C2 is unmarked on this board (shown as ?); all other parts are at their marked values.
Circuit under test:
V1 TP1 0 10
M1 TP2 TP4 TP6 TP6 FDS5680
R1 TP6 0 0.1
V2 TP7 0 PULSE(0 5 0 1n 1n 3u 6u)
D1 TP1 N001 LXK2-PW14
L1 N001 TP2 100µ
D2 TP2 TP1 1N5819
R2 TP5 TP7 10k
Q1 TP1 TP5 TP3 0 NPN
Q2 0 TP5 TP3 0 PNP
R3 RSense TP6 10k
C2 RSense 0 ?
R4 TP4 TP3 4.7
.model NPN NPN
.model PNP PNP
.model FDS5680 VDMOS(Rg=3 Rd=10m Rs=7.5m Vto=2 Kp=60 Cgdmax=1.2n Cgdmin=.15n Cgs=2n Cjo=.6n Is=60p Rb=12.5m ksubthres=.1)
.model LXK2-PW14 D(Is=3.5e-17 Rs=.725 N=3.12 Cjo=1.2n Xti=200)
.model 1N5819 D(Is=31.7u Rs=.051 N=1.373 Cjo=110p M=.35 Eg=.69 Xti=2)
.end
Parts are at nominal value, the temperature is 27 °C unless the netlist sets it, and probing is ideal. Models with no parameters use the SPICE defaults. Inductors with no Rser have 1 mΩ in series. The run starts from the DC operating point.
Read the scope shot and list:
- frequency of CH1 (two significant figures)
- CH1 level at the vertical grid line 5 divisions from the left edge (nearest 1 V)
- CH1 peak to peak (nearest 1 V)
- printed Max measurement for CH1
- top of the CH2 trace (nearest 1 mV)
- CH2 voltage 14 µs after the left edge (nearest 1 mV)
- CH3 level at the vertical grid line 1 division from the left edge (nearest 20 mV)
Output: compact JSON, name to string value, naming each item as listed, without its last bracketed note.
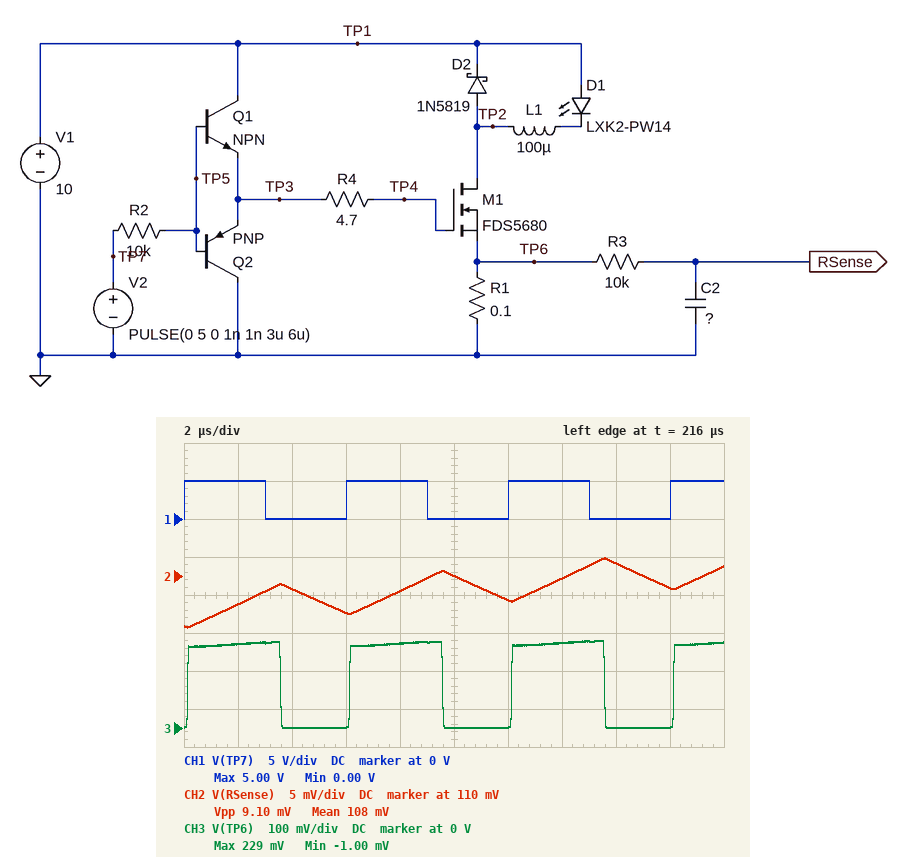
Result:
{"frequency of CH1": "170 kHz", "CH1 level at the vertical grid line 5 divisions from the left edge": "0 V", "CH1 peak to peak": "5 V", "printed Max measurement for CH1": "5.00 V", "top of the CH2 trace": "112 mV", "CH2 voltage 14 µs after the left edge": "110 mV", "CH3 level at the vertical grid line 1 division from the left edge": "220 mV"}
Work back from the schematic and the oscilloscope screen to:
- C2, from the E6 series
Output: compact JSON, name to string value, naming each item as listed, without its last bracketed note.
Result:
{"C2, from the E6 series": "6.8 nF"}
